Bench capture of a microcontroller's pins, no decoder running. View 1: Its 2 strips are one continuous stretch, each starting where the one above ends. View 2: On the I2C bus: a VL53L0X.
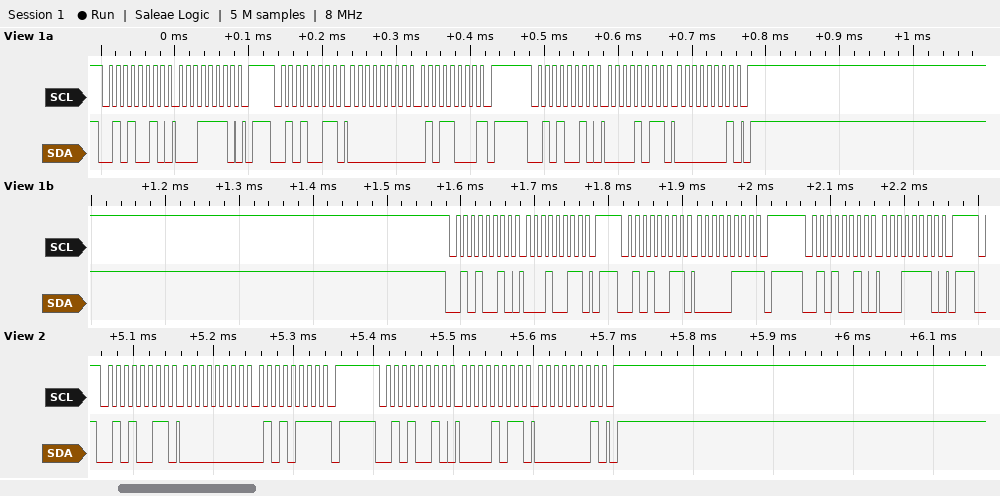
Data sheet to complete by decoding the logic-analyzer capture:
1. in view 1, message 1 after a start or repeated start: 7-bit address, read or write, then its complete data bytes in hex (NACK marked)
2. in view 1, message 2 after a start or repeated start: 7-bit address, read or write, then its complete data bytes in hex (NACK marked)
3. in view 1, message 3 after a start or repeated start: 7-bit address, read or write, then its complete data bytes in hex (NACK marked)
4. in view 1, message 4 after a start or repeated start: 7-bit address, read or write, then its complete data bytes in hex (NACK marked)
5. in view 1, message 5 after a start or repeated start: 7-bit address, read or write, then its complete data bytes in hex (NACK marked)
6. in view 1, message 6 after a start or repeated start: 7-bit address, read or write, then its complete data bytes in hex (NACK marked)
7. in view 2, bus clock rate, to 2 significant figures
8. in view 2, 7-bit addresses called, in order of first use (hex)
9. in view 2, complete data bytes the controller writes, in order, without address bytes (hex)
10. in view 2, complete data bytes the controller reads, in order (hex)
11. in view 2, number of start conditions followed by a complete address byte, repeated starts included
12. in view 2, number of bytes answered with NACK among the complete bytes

0x29 write: 1E
0x29 read: 00 58 NACK
0x29 write: 0B 01
0x29 write: 13
0x29 read: 07 NACK
0x29 write: 1E
100 kHz
0x29
0B 01
00 57
2
1
